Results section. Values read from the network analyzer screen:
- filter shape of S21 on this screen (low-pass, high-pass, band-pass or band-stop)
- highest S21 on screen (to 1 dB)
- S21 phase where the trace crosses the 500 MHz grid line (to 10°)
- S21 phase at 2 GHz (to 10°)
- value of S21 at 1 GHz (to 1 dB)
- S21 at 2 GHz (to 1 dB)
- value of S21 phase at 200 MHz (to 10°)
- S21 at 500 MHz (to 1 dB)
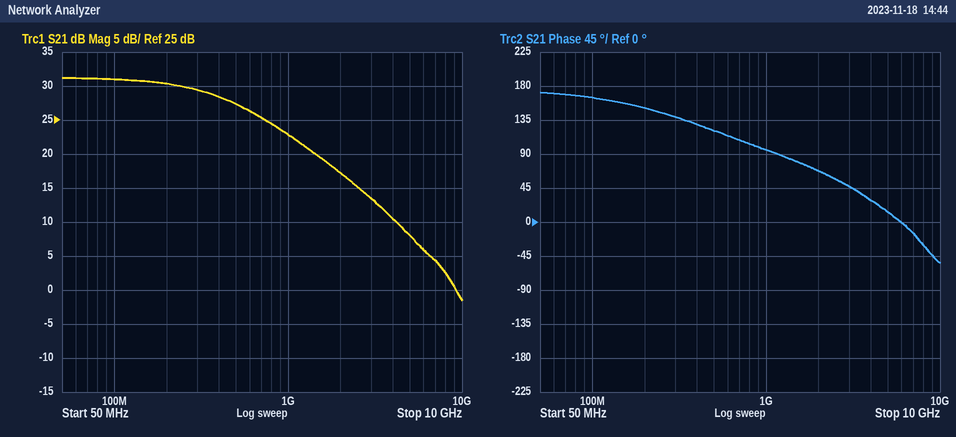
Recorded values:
low-pass
31 dB
120°
70°
23 dB
17 dB
150°
27 dB
